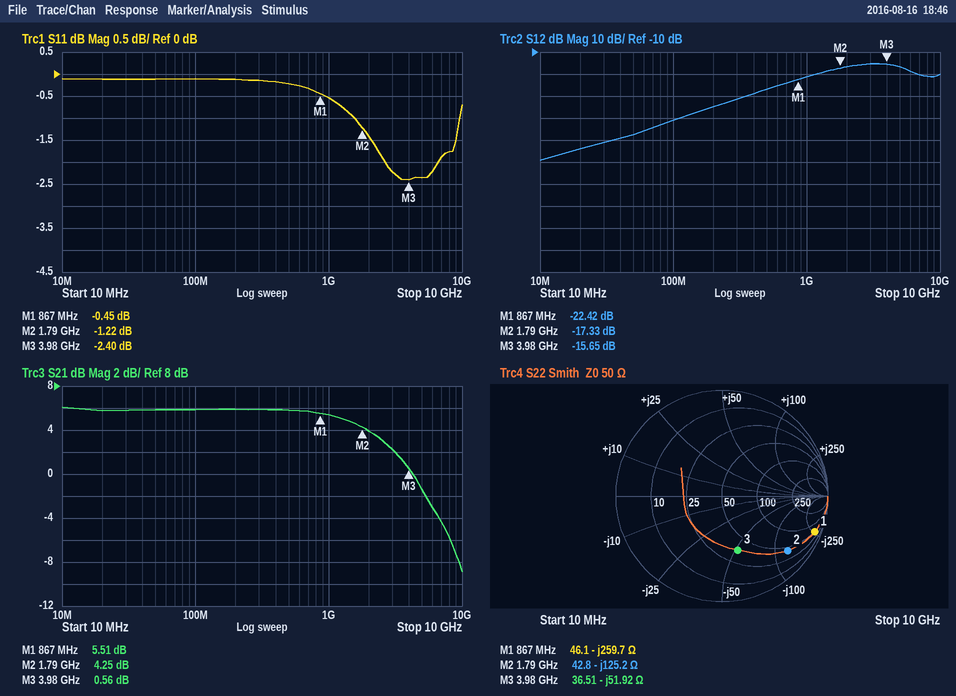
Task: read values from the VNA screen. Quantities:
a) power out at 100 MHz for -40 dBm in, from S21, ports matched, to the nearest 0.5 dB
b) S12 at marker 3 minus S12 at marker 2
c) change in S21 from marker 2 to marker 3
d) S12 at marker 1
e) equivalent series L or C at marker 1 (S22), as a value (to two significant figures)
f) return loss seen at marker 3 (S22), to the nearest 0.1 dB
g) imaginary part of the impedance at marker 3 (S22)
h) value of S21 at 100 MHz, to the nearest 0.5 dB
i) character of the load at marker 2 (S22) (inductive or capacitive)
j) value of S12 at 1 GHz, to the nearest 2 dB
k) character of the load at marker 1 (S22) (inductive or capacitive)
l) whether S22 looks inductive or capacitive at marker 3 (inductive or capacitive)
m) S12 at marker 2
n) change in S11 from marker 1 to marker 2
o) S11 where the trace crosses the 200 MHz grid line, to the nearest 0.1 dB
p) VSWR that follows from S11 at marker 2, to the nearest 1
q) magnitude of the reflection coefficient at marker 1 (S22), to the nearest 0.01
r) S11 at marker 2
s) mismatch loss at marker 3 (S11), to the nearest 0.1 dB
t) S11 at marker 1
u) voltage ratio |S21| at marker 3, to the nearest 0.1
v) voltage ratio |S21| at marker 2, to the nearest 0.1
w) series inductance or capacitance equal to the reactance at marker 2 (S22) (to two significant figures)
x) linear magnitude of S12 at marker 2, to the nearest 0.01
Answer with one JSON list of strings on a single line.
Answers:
["-34.0 dBm", "1.68 dB", "-3.69 dB", "-22.42 dB", "710 fF", "5.5 dB", "-51.92 Ω", "6.0 dB", "capacitive", "-22 dB", "capacitive", "capacitive", "-17.33 dB", "-0.77 dB", "-0.1 dB", "14", "0.94", "-1.22 dB", "3.7 dB", "-0.45 dB", "1.1", "1.6", "710 fF", "0.14"]
